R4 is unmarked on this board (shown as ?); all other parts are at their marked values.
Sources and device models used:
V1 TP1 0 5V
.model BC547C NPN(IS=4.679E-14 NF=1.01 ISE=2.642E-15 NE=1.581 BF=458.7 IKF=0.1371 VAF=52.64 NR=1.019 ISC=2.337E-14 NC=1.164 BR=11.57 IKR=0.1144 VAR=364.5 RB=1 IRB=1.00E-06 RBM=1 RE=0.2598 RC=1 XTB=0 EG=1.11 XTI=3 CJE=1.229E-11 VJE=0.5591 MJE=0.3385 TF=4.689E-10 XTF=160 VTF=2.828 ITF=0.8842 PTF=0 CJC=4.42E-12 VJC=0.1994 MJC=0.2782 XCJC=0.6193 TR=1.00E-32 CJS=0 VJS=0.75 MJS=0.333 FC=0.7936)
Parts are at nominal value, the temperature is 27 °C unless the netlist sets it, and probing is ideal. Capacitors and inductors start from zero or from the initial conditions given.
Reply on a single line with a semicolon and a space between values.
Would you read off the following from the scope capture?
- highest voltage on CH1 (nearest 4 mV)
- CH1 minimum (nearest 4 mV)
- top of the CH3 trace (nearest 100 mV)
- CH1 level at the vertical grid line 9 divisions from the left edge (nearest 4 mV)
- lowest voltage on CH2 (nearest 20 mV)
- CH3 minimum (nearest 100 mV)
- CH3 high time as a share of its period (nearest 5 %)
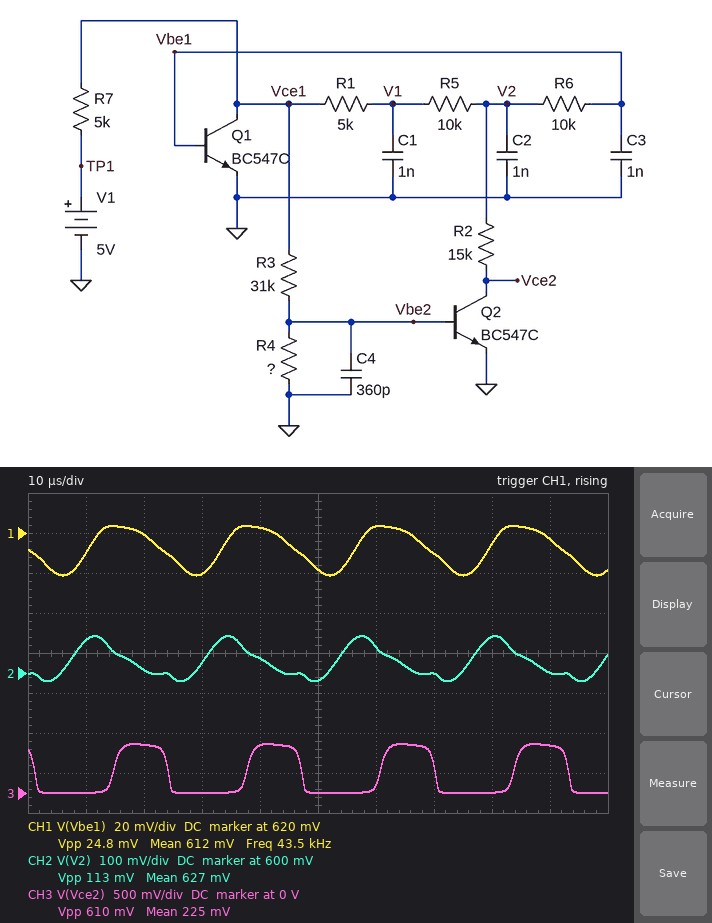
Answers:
624 mV; 600 mV; 600 mV; 616 mV; 580 mV; 0 V; 40 %
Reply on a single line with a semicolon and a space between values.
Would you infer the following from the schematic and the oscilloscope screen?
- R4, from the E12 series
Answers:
150 kΩ
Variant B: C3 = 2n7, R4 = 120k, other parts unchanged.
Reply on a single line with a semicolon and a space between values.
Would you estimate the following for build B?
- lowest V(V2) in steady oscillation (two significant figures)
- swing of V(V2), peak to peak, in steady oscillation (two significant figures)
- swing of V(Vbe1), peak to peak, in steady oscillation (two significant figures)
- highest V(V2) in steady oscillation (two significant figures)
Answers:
550 mV; 160 mV; 20 mV; 710 mV
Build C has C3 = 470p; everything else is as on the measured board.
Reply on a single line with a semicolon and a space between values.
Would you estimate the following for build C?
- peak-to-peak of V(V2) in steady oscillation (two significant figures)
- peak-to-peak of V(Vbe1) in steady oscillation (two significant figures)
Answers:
96 mV; 28 mV
